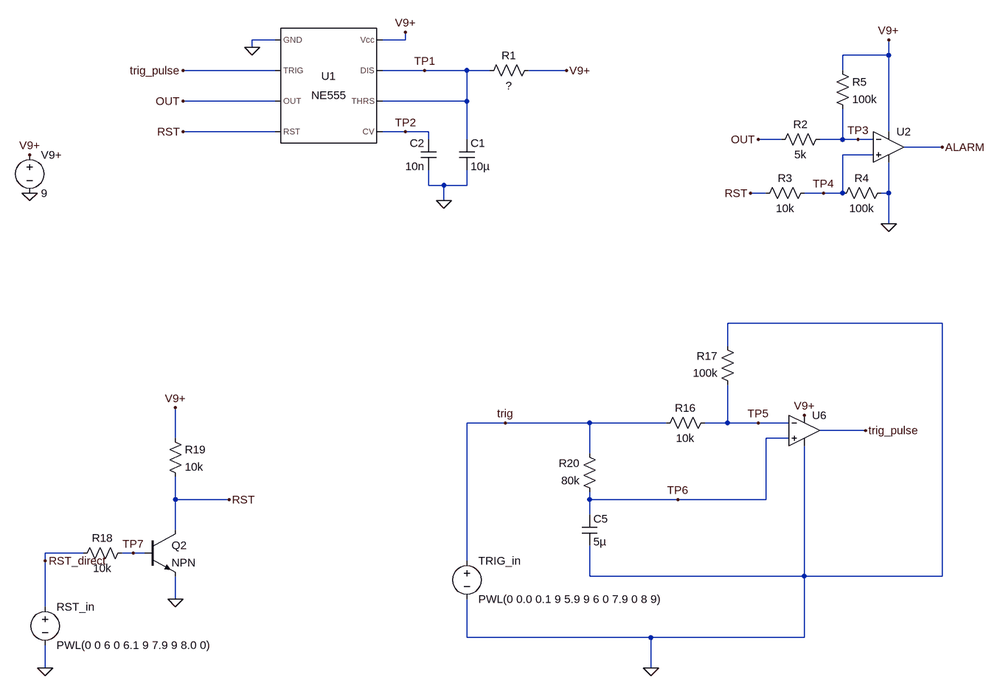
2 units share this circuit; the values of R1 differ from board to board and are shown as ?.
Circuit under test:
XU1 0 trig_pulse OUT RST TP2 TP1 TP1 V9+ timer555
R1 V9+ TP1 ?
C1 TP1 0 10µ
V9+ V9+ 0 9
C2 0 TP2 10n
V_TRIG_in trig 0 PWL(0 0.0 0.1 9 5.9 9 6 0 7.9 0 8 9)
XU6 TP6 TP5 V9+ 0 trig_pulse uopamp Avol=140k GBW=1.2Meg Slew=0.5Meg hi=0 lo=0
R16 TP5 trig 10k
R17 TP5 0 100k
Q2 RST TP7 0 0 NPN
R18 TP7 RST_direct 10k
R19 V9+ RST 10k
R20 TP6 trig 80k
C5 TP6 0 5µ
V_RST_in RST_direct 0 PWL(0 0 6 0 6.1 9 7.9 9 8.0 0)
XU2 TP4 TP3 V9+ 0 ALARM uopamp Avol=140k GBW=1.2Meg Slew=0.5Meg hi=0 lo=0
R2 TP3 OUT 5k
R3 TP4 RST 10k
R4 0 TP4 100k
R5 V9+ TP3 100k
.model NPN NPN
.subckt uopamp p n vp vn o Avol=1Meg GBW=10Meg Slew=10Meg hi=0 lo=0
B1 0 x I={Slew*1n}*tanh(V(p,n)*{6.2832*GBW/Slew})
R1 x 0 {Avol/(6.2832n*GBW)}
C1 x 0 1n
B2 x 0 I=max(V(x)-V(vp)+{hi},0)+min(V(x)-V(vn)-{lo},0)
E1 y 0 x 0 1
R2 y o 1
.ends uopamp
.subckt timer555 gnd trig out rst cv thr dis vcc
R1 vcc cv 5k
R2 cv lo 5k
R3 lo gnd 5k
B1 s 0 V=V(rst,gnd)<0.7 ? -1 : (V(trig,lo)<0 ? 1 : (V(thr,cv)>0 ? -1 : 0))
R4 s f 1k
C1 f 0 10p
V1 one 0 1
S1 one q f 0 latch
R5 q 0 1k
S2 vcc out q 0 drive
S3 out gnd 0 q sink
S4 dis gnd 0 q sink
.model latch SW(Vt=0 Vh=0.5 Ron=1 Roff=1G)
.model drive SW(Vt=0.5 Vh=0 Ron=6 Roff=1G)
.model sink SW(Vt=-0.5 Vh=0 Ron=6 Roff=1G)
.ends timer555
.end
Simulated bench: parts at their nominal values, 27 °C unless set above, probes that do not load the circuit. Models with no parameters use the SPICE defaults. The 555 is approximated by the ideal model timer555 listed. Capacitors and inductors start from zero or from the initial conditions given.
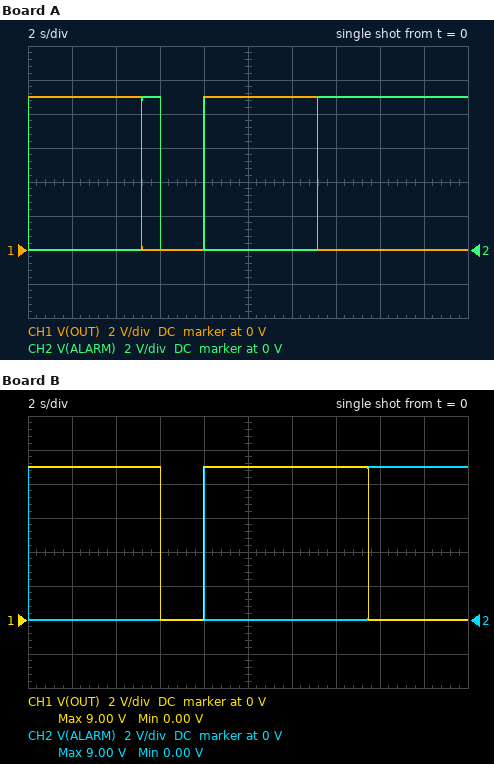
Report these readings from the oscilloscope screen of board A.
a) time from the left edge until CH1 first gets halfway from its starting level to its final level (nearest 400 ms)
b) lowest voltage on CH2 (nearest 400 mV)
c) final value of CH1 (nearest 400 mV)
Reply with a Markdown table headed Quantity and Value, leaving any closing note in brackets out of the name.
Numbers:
| Quantity | Value |
|---|---|
| time from the left edge until CH1 first gets halfway from its starting level to its final level | 5.2 s |
| lowest voltage on CH2 | 0 V |
| final value of CH1 | 0 V |
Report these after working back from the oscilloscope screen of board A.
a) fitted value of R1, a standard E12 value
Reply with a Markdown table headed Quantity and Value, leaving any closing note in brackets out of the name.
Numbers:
| Quantity | Value |
|---|---|
| fitted value of R1, a standard E12 value | 470 kΩ |
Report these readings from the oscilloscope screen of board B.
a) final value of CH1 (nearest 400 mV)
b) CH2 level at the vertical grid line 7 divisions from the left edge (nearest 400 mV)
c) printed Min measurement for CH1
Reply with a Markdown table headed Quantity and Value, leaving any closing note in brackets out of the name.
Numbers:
| Quantity | Value |
|---|---|
| final value of CH1 | 0 V |
| CH2 level at the vertical grid line 7 divisions from the left edge | 0 V |
| printed Min measurement for CH1 | 0.00 V |
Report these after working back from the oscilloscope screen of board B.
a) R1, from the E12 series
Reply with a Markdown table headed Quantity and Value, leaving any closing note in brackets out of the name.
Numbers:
| Quantity | Value |
|---|---|
| R1, from the E12 series | 680 kΩ |
